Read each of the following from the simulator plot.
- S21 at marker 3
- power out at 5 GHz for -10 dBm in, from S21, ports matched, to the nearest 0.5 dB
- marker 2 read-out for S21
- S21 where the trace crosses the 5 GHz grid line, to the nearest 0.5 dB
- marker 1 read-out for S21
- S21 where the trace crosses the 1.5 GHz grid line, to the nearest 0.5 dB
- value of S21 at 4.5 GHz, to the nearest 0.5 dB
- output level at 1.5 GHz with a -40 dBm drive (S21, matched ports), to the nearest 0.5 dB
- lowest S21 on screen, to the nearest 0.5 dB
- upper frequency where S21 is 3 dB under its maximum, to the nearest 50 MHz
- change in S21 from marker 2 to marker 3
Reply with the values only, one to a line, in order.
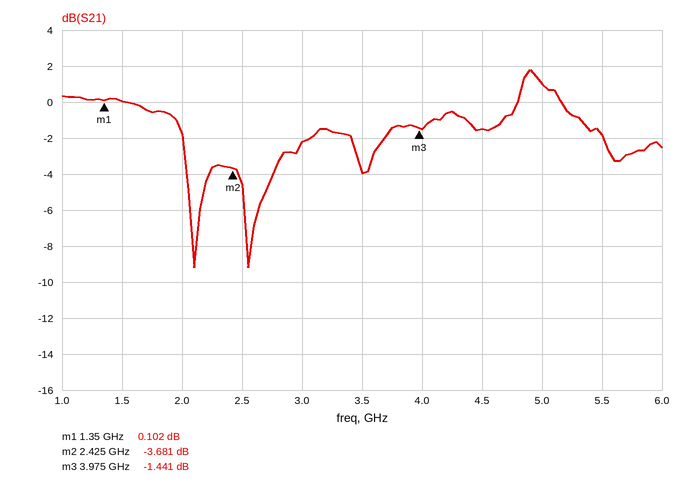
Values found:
-1.441 dB
-9.0 dBm
-3.681 dB
1.0 dB
0.102 dB
0.0 dB
-1.5 dB
-40.0 dBm
-9.0 dB
5.35 GHz
2.240 dB
